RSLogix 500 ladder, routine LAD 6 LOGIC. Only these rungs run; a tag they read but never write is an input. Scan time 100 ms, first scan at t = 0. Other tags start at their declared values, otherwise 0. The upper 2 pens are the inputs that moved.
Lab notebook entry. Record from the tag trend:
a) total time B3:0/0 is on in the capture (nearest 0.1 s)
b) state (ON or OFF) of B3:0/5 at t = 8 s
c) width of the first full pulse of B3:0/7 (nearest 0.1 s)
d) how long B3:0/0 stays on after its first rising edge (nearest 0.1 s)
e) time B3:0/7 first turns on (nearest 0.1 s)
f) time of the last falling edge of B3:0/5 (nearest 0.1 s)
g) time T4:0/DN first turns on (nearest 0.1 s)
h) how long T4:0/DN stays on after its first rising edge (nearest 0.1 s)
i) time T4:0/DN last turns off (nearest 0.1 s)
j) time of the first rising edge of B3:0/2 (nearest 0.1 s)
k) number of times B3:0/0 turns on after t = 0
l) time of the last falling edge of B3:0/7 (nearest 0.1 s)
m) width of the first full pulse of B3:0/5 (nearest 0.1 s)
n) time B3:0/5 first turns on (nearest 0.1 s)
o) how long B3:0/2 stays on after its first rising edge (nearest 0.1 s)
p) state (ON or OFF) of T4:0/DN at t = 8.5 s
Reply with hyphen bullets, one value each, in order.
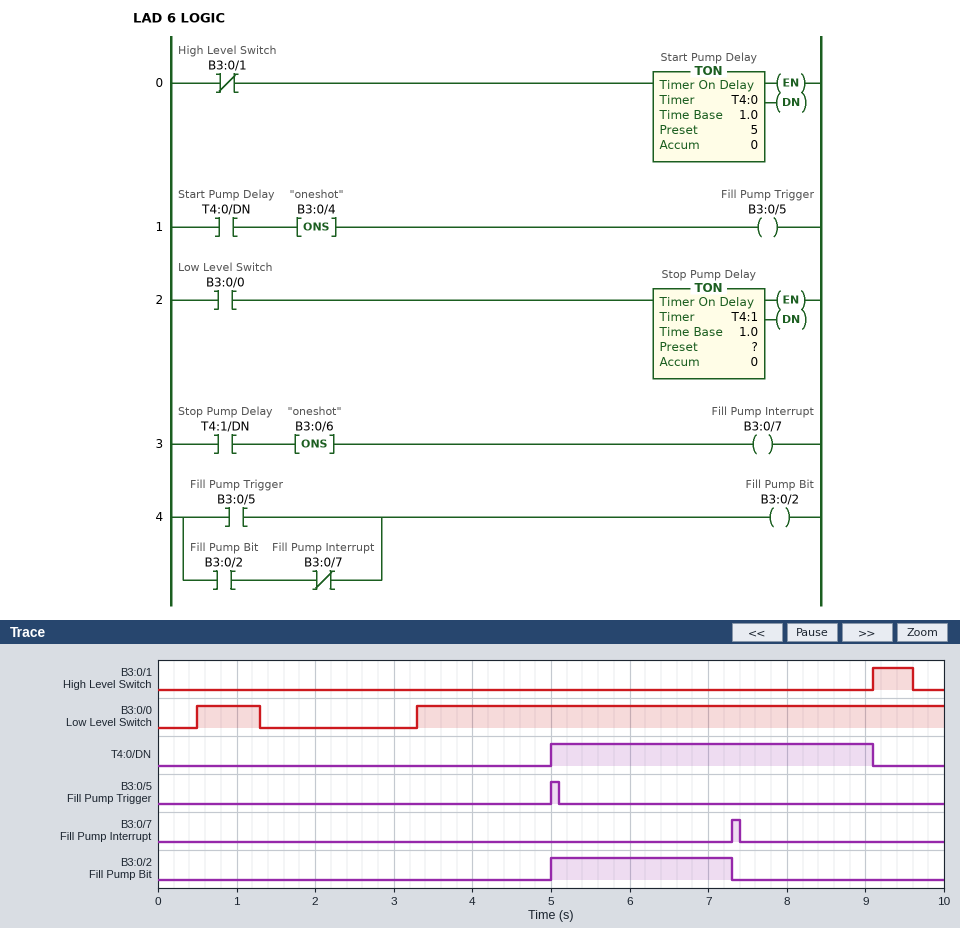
- 7.5 s
- OFF
- 0.1 s
- 0.8 s
- 7.3 s
- 5.1 s
- 5.0 s
- 4.1 s
- 9.1 s
- 5.0 s
- 2
- 7.4 s
- 0.1 s
- 5.0 s
- 2.3 s
- ON
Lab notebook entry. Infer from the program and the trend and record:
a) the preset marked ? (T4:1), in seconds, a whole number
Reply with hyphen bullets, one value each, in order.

- 4 s
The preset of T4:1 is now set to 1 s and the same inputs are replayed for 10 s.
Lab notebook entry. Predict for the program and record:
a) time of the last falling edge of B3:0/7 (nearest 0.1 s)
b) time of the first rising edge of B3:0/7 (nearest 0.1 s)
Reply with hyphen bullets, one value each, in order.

- 4.4 s
- 4.3 s
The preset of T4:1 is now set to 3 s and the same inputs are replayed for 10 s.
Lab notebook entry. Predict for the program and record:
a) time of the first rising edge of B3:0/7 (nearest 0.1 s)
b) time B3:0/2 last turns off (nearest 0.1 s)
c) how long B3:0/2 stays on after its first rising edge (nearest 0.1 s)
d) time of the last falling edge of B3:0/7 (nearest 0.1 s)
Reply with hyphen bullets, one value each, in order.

- 6.3 s
- 6.3 s
- 1.3 s
- 6.4 s
